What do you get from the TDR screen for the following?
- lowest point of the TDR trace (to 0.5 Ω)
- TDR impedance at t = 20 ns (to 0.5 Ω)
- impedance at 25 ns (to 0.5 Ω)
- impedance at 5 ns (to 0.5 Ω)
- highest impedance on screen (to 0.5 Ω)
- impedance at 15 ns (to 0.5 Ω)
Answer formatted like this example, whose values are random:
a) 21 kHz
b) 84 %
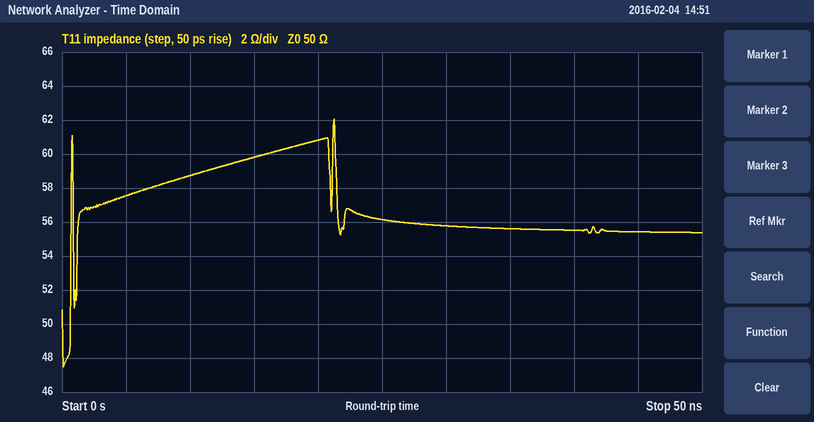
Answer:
a) 47.5 Ω
b) 61.0 Ω
c) 56.0 Ω
d) 57.5 Ω
e) 62.0 Ω
f) 60.0 Ω
